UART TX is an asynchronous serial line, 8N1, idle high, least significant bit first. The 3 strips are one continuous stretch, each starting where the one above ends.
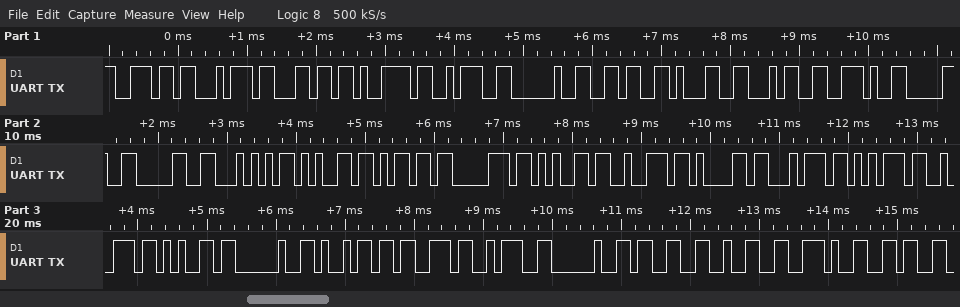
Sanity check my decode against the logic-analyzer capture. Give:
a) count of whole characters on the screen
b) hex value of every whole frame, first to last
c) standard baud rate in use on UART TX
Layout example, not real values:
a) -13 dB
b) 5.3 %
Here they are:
a) 32
b) 0x6E 0x74 0x6C 0x79 0x3A 0x20 0x36 0x31 0x34 0x2E 0x30 0x30 0x54 0x65 0x6D 0x70 0x65 0x72 0x61 0x74 0x75 0x72 0x65 0x20 0x69 0x73 0x3A 0x20 0x33 0x32 0x2E 0x36
c) 9600 baud
